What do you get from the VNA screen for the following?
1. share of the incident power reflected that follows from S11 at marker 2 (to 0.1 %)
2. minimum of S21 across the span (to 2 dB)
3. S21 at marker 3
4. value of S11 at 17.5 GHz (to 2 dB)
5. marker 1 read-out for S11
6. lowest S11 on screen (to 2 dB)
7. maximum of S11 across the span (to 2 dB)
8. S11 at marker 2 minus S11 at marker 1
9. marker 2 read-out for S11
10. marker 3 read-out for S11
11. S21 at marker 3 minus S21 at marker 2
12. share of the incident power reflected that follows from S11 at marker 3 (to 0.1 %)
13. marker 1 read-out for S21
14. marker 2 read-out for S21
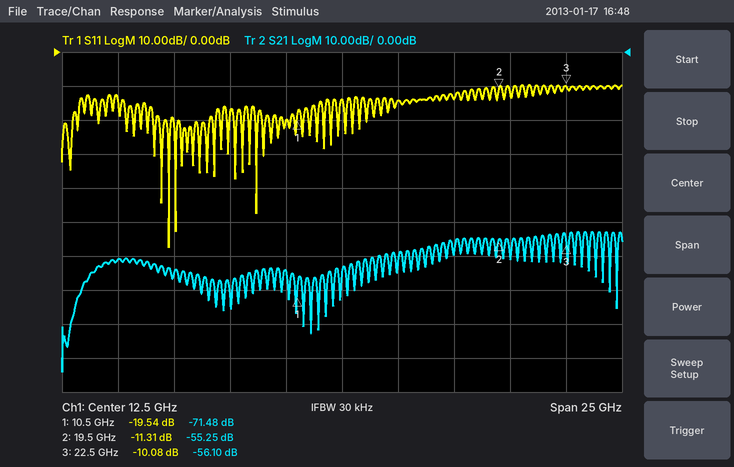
7.4 %
-94 dB
-56.10 dB
-14 dB
-19.54 dB
-58 dB
-10 dB
8.23 dB
-11.31 dB
-10.08 dB
-0.85 dB
9.8 %
-71.48 dB
-55.25 dB
